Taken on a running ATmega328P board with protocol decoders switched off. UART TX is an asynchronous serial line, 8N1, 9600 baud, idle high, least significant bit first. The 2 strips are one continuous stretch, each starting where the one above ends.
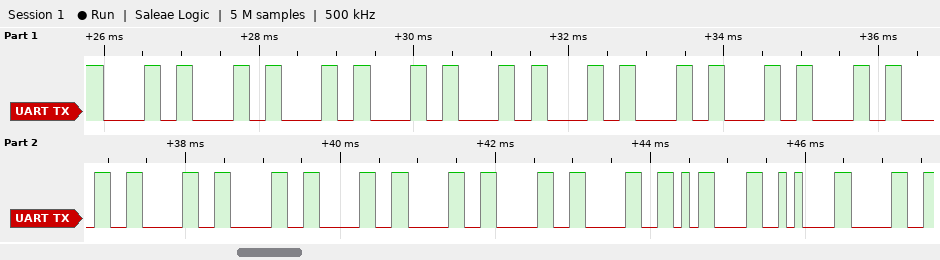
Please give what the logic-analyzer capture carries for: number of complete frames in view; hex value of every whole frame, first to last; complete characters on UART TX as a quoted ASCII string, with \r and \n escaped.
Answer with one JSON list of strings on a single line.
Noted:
["19", "30 30 30 30 30 30 30 30 30 30 30 30 30 30 30 30 0D 0A 30", "\"0000000000000000\\r\\n0\""]
